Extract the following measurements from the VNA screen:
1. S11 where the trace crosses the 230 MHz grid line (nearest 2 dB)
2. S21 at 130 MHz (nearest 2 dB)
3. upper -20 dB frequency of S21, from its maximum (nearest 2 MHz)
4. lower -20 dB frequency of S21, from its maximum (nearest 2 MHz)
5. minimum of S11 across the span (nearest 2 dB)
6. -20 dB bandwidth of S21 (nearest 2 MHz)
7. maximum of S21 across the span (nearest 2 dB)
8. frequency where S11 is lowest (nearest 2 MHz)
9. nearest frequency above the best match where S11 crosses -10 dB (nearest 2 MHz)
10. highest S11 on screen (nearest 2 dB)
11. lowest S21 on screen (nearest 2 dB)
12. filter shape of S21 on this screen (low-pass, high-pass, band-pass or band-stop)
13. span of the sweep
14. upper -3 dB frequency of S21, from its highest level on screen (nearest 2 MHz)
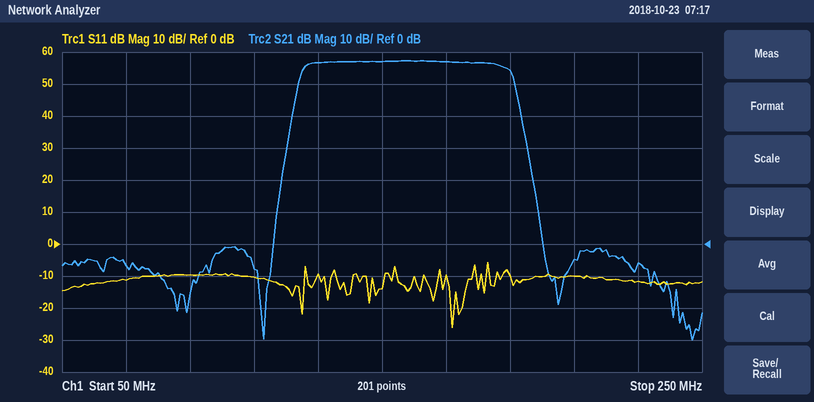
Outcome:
-12 dB
56 dB
194 MHz
122 MHz
-26 dB
72 MHz
58 dB
172 MHz
178 MHz
-6 dB
-30 dB
band-pass
200 MHz
190 MHz
